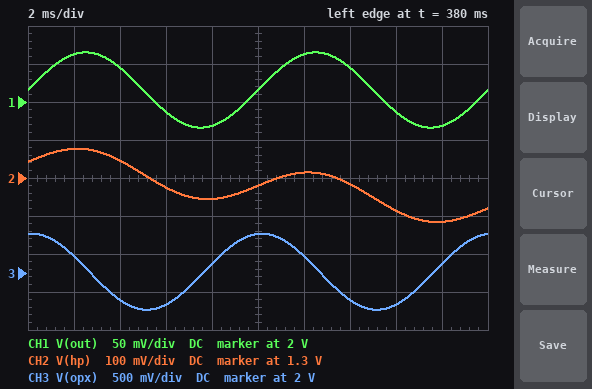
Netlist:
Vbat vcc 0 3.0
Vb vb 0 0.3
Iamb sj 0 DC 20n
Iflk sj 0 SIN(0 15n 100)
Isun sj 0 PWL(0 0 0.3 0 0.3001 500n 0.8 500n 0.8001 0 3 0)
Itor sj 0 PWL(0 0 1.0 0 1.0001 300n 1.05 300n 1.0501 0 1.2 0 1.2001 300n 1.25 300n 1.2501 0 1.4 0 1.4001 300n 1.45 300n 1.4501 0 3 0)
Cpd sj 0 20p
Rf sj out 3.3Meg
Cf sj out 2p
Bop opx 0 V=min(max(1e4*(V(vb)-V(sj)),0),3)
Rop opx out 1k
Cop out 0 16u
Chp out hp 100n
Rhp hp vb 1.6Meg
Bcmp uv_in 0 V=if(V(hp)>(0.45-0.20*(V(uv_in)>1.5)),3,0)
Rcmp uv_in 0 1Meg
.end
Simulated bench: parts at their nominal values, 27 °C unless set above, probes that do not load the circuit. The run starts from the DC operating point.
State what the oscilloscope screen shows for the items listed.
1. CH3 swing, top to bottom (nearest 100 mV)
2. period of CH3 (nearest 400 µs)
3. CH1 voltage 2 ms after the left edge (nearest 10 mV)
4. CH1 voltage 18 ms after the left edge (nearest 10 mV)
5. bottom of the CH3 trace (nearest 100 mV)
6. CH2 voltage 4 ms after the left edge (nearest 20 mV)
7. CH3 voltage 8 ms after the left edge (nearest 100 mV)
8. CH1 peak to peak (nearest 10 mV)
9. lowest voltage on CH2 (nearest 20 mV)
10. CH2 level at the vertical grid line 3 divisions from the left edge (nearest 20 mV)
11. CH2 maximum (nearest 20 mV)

1.0 V
10.0 ms
2.06 V
1.97 V
1.5 V
1.34 V
2.1 V
100 mV
1.18 V
1.28 V
1.38 V
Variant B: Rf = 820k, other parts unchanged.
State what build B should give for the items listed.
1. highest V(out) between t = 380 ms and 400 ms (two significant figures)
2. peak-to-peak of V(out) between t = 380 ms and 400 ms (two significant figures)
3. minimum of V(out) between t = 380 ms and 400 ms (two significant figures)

740 mV
25 mV
710 mV
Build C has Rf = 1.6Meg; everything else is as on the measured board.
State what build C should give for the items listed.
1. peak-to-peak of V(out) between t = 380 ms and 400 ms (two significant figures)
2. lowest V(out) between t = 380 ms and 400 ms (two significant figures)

48 mV
1.1 V
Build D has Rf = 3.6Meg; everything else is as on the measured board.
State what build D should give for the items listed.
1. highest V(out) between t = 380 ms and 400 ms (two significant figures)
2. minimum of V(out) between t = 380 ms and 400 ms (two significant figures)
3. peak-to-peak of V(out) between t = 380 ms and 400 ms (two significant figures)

2.2 V
2.1 V
110 mV
